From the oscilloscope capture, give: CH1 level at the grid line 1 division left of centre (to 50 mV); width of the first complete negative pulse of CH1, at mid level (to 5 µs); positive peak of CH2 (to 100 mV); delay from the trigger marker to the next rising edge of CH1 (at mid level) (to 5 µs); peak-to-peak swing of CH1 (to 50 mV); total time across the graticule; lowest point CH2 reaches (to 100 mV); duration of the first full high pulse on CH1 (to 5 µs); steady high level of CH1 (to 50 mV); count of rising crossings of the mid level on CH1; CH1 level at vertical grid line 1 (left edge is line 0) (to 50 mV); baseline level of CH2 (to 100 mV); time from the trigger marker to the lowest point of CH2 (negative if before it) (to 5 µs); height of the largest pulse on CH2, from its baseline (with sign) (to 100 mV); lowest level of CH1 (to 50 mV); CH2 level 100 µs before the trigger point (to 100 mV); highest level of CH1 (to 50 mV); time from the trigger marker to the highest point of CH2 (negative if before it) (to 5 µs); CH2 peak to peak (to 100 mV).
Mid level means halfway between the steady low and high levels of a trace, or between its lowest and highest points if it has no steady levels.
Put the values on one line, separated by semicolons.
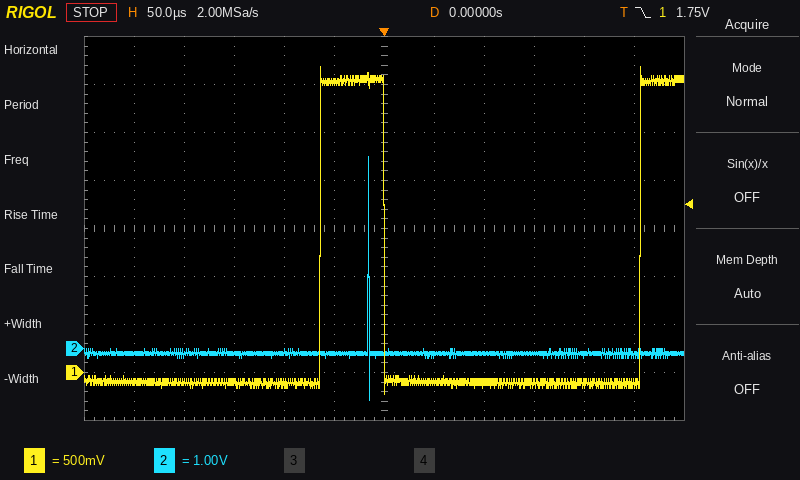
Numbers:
3.05 V; 255 µs; 4.0 V; 255 µs; 3.40 V; 600 µs; -1.1 V; 65 µs; 3.05 V; 2; -100 mV; -100 mV; -15 µs; +4.1 V; -200 mV; -100 mV; 3.20 V; -15 µs; 5.1 V
